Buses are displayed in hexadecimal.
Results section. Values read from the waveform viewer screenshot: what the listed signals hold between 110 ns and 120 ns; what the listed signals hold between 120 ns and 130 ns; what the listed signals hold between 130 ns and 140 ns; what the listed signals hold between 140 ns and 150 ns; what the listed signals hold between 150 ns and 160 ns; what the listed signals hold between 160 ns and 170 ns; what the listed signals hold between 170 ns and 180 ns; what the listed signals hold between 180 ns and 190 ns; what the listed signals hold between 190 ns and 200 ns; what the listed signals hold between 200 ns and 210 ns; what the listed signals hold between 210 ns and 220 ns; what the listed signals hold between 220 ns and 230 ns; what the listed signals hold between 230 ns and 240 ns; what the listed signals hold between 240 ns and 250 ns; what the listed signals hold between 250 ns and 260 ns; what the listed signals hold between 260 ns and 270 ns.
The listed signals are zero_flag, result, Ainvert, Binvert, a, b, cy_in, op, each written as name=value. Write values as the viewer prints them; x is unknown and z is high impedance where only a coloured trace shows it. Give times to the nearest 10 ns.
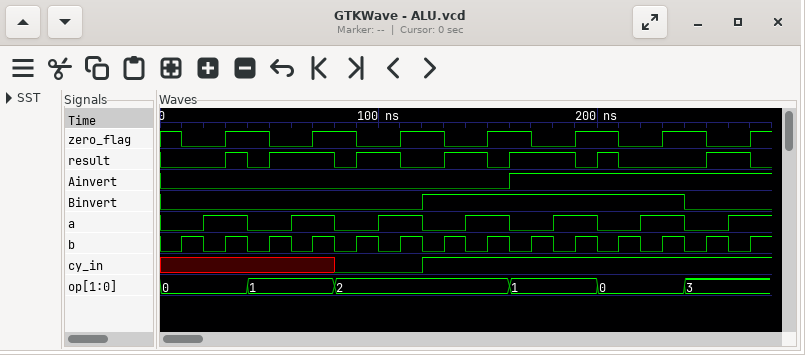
zero_flag=1, result=0, Ainvert=0, Binvert=0, a=1, b=1, cy_in=0, op=2
zero_flag=1, result=0, Ainvert=0, Binvert=1, a=0, b=0, cy_in=1, op=2
zero_flag=0, result=1, Ainvert=0, Binvert=1, a=0, b=1, cy_in=1, op=2
zero_flag=0, result=1, Ainvert=0, Binvert=1, a=1, b=0, cy_in=1, op=2
zero_flag=1, result=0, Ainvert=0, Binvert=1, a=1, b=1, cy_in=1, op=2
zero_flag=1, result=1, Ainvert=1, Binvert=1, a=0, b=0, cy_in=1, op=1
zero_flag=0, result=1, Ainvert=1, Binvert=1, a=0, b=1, cy_in=1, op=1
zero_flag=0, result=1, Ainvert=1, Binvert=1, a=1, b=0, cy_in=1, op=1
zero_flag=1, result=0, Ainvert=1, Binvert=1, a=1, b=1, cy_in=1, op=1
zero_flag=1, result=1, Ainvert=1, Binvert=1, a=0, b=0, cy_in=1, op=0
zero_flag=0, result=0, Ainvert=1, Binvert=1, a=0, b=1, cy_in=1, op=0
zero_flag=0, result=0, Ainvert=1, Binvert=1, a=1, b=0, cy_in=1, op=0
zero_flag=1, result=0, Ainvert=1, Binvert=1, a=1, b=1, cy_in=1, op=0
zero_flag=1, result=0, Ainvert=1, Binvert=0, a=0, b=0, cy_in=1, op=3
zero_flag=0, result=1, Ainvert=1, Binvert=0, a=0, b=1, cy_in=1, op=3
zero_flag=0, result=1, Ainvert=1, Binvert=0, a=1, b=0, cy_in=1, op=3
